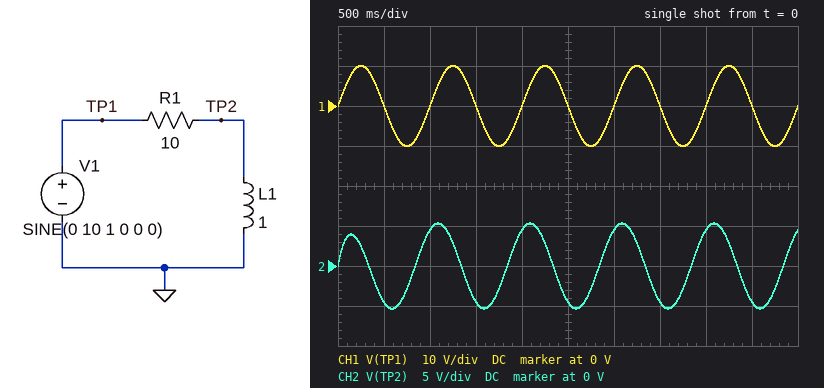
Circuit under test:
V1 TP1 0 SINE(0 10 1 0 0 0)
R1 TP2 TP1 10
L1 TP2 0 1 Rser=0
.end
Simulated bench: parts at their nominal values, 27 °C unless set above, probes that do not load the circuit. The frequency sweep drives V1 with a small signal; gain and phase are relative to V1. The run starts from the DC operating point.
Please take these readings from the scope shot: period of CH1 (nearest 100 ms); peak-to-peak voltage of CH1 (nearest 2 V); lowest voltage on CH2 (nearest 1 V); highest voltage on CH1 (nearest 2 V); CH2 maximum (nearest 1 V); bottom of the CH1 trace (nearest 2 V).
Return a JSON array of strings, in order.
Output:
["1.0 s", "20 V", "-5 V", "10 V", "5 V", "-10 V"]
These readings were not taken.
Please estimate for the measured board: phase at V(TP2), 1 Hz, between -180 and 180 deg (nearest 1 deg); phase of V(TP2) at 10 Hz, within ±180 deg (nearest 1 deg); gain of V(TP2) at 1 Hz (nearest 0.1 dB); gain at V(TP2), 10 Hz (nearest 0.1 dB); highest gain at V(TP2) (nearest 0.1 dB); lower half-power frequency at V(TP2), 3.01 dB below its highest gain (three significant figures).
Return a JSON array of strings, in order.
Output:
["58 deg", "9 deg", "-5.5 dB", "-0.1 dB", "0 dB", "1.59 Hz"]
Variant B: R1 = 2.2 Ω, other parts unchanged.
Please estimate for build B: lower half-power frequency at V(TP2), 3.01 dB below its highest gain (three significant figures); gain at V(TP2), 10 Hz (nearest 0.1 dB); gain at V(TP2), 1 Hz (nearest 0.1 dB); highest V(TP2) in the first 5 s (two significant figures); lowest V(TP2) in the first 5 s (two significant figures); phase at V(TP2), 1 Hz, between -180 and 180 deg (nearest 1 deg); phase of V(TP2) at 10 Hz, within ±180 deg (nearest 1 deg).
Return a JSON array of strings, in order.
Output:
["350 mHz", "0 dB", "-0.5 dB", "9.4 V", "-10 V", "19 deg", "2 deg"]
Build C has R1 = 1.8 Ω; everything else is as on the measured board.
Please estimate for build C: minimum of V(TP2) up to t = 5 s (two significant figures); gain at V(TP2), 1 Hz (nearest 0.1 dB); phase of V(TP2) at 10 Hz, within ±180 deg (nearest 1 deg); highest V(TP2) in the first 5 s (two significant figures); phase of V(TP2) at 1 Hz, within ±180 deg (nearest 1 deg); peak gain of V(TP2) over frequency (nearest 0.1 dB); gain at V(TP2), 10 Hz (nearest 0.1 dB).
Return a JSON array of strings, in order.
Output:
["-10 V", "-0.3 dB", "2 deg", "9.6 V", "16 deg", "0 dB", "0 dB"]
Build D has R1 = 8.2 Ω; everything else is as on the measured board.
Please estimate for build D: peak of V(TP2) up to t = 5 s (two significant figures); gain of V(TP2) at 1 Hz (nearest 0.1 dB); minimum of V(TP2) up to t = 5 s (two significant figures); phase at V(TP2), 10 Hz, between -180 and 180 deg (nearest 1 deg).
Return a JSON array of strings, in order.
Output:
["6.1 V", "-4.3 dB", "-6.1 V", "7 deg"]
